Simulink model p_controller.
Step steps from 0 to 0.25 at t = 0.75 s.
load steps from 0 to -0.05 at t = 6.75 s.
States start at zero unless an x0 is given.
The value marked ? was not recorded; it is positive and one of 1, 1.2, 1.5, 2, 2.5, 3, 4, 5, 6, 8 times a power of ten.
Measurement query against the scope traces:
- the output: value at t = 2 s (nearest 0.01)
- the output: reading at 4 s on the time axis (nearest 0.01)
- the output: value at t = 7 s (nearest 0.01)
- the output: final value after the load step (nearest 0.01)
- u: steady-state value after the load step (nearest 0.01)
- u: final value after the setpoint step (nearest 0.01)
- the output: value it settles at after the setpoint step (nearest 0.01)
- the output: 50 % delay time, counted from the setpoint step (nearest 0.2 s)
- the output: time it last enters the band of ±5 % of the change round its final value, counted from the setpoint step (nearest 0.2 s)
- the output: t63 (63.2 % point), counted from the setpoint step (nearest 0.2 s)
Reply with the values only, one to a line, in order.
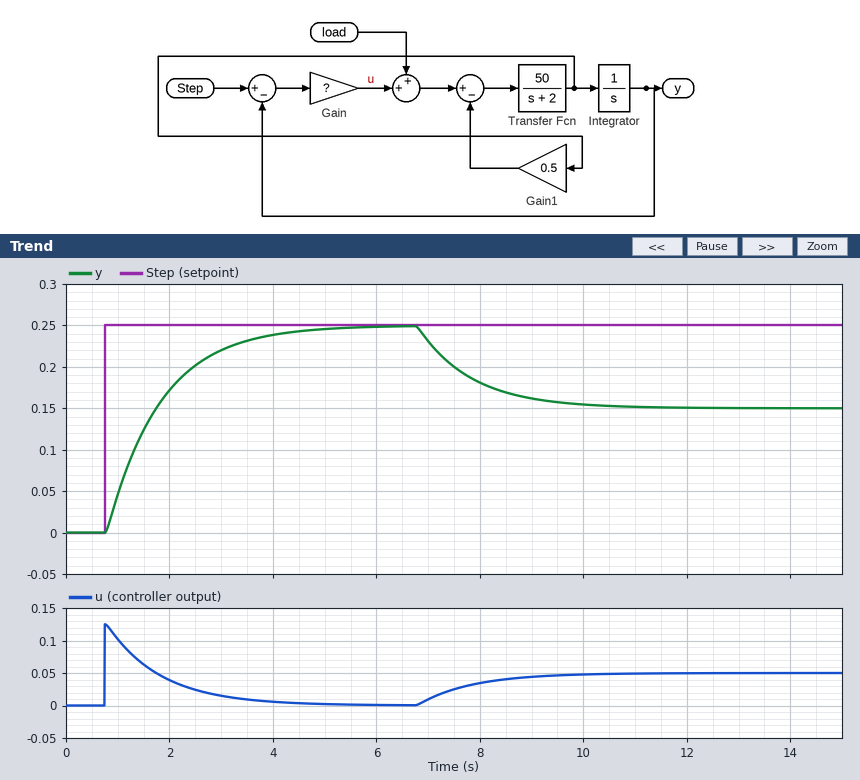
0.17
0.24
0.23
0.15
0.05
0.00
0.25
0.8 s
3.2 s
1.0 s
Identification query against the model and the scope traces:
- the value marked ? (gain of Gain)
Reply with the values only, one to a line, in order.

0.5
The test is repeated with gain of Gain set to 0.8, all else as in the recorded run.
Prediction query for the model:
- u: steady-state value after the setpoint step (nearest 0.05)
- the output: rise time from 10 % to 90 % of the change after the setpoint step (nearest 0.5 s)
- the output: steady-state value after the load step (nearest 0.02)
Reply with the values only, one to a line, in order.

0.00
1.5 s
0.18
